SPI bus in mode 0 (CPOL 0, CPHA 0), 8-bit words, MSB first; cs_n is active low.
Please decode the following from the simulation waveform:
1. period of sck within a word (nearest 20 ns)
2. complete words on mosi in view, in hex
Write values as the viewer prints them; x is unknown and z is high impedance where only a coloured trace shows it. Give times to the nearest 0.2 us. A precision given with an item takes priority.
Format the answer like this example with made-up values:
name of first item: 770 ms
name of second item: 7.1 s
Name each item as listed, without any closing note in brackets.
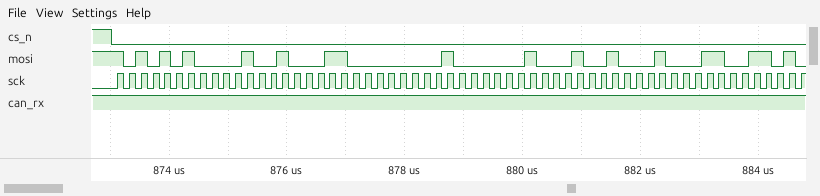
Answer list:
period of sck within a word: 200 ns
complete words on mosi in view, in hex: AA, 12, 30, 08, 11, 22, 33
